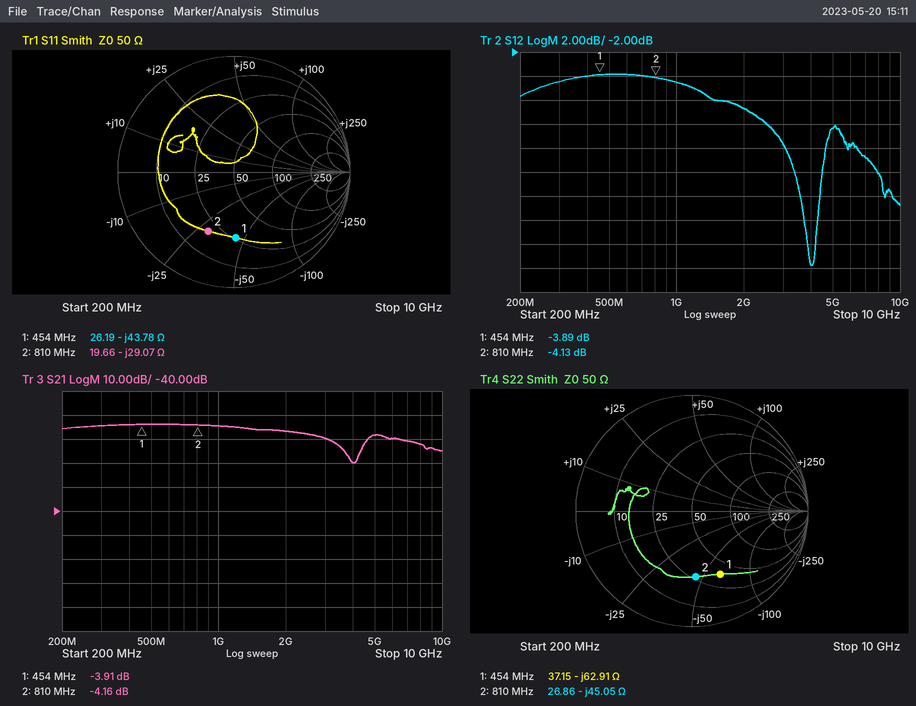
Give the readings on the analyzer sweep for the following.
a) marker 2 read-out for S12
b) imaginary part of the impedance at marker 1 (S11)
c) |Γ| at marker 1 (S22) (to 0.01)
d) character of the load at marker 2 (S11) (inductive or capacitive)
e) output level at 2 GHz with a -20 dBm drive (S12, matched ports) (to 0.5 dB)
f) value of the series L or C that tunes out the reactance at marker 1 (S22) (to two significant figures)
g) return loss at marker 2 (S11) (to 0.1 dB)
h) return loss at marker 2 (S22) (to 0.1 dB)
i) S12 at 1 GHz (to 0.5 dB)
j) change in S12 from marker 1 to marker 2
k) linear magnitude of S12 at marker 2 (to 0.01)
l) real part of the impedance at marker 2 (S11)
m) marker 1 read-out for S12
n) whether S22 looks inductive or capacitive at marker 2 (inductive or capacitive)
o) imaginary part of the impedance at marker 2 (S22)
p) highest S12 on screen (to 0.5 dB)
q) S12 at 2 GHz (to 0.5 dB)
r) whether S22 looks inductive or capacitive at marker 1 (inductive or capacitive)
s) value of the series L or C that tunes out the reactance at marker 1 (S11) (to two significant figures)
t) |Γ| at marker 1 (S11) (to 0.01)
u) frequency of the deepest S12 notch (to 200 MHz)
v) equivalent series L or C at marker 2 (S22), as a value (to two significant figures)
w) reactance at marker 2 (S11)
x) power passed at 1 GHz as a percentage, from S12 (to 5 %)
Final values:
-4.13 dB
-43.78 Ω
0.60
capacitive
-26.5 dBm
22 nH
5.1 dB
4.9 dB
-4.5 dB
-0.24 dB
0.62
19.66 Ω
-3.89 dB
capacitive
-45.05 Ω
-4.0 dB
-6.5 dB
capacitive
15 nH
0.57
4.0 GHz
4.4 pF
-29.07 Ω
35 %
